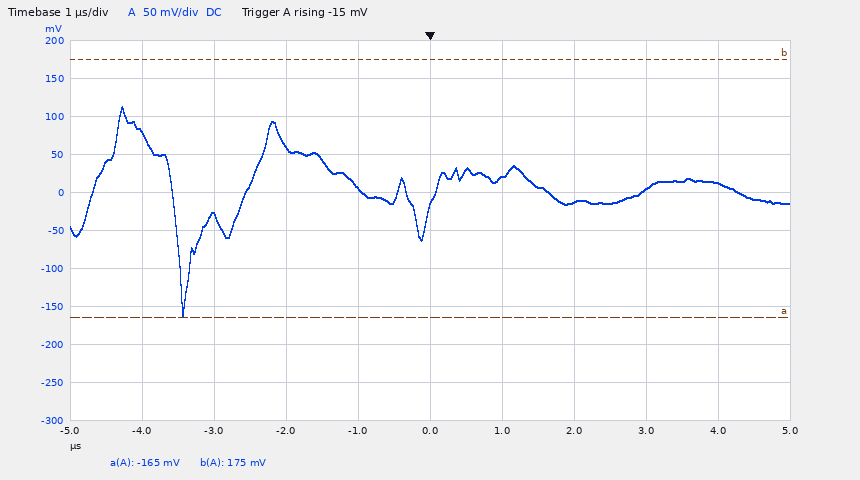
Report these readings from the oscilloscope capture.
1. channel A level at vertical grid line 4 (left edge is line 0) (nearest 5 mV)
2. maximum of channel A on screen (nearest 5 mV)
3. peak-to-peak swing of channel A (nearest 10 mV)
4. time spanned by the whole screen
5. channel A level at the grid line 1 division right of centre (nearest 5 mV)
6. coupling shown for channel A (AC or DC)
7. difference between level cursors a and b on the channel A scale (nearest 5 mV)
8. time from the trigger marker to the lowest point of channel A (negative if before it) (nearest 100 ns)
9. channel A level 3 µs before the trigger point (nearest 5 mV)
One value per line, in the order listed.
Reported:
5 mV
115 mV
280 mV
10 µs
20 mV
DC
340 mV
-3.4 µs
-30 mV
